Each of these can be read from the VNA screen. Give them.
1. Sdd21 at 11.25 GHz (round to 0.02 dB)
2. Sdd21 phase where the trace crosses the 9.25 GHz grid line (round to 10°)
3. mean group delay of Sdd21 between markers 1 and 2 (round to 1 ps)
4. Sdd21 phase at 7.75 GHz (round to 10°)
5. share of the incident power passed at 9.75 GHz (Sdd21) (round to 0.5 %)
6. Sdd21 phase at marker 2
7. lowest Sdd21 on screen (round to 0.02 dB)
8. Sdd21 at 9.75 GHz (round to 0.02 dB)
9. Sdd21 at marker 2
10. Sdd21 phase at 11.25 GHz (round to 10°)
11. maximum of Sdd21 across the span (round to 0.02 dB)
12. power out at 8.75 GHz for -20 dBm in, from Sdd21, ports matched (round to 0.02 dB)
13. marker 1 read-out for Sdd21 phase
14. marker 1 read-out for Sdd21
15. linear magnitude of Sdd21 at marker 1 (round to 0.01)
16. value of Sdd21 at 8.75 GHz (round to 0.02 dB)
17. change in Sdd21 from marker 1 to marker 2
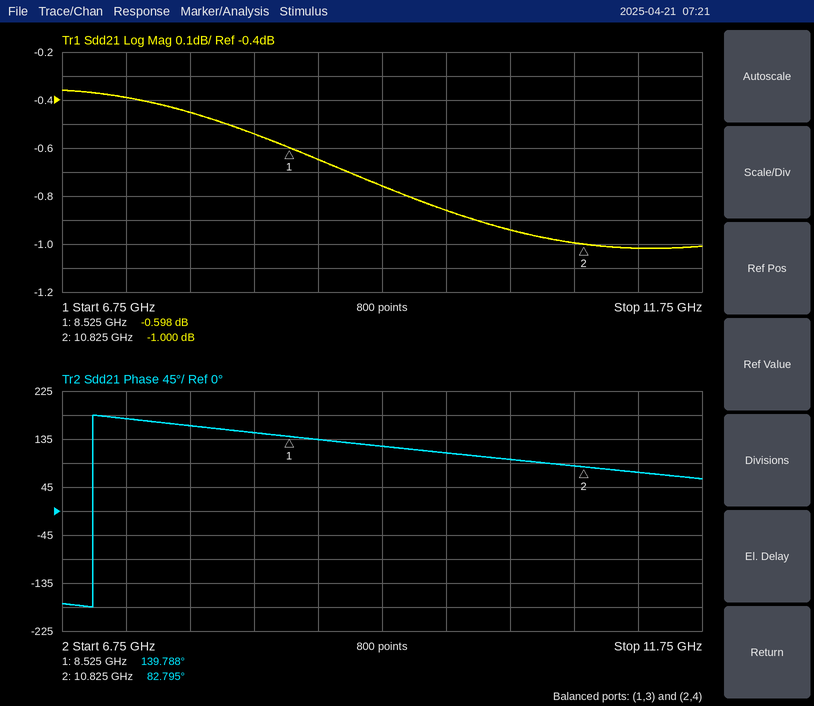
-1.02 dB
120°
69 ps
160°
82.0 %
82.795°
-1.02 dB
-0.86 dB
-1.000 dB
70°
-0.36 dB
-20.64 dBm
139.788°
-0.598 dB
0.93
-0.64 dB
-0.402 dB
